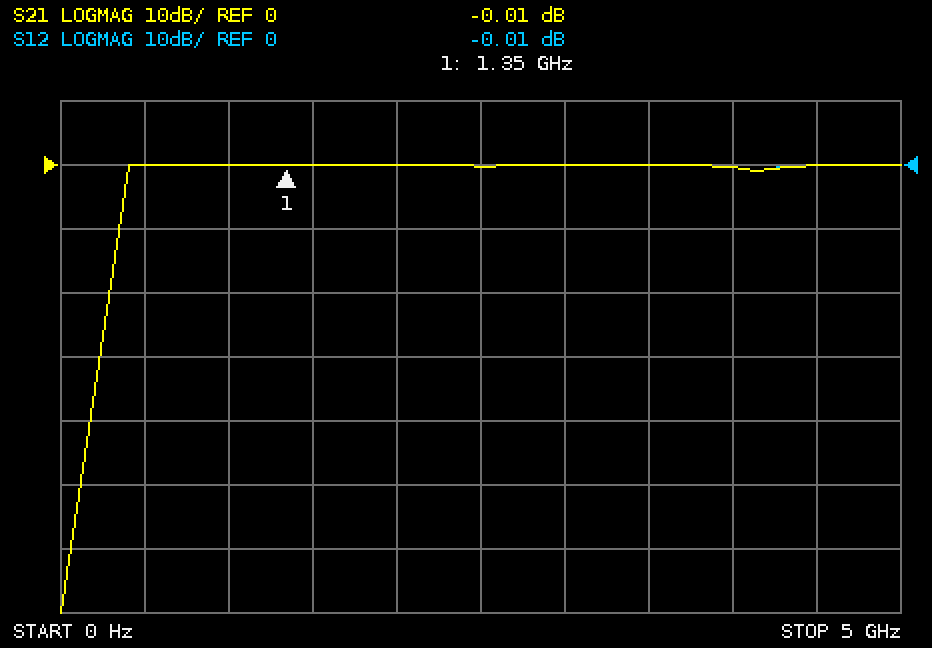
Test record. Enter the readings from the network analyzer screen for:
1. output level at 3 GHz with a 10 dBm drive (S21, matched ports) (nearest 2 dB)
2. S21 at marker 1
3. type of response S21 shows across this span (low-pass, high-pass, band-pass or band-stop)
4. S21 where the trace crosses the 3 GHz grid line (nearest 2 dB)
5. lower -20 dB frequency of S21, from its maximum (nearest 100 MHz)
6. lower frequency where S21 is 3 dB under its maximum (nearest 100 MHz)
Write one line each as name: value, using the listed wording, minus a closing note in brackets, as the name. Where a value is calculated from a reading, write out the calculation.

output level at 3 GHz with a 10 dBm drive (S21, matched ports): 10 dBm + (0 dB) = 10 dBm
S21 at marker 1: -0.01 dB
type of response S21 shows across this span: high-pass
S21 where the trace crosses the 3 GHz grid line: 0 dB
lower -20 dB frequency of S21, from its maximum: 300 MHz
lower frequency where S21 is 3 dB under its maximum: 400 MHz
